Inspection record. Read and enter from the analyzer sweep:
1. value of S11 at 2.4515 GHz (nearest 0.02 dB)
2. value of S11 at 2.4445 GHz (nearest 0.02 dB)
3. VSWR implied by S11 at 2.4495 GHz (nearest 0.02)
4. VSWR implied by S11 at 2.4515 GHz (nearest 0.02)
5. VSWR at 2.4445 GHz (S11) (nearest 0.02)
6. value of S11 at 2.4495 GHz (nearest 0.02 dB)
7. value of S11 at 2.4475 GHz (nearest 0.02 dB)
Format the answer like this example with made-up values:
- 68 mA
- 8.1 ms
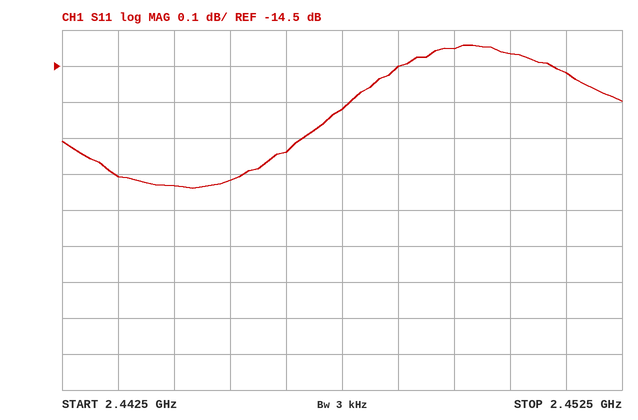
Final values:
- -14.52 dB
- -14.84 dB
- 1.46
- 1.46
- 1.44
- -14.46 dB
- -14.62 dB
